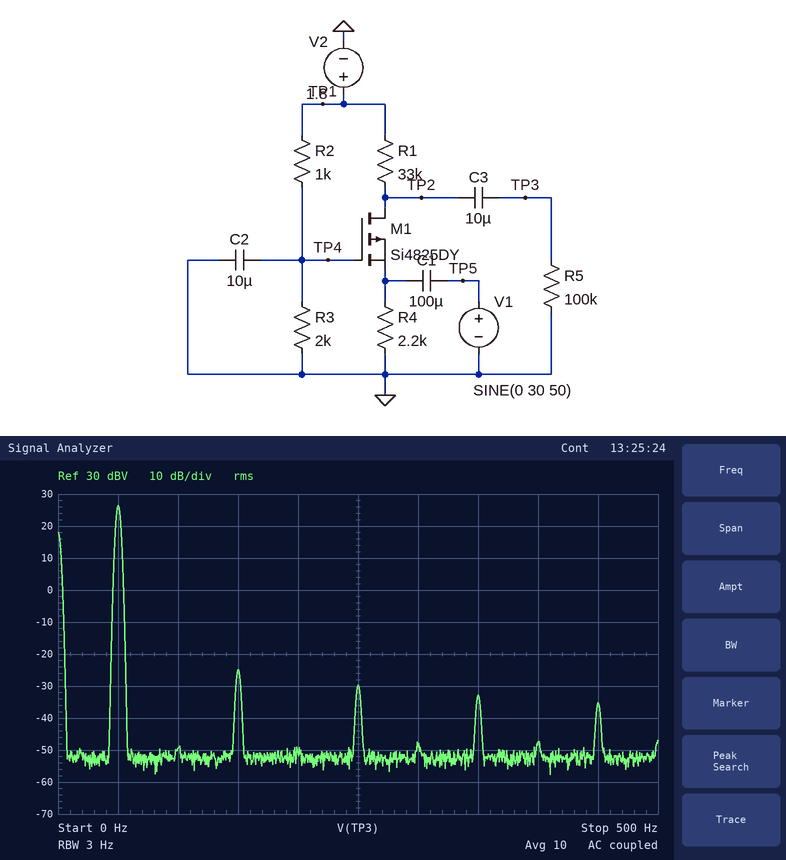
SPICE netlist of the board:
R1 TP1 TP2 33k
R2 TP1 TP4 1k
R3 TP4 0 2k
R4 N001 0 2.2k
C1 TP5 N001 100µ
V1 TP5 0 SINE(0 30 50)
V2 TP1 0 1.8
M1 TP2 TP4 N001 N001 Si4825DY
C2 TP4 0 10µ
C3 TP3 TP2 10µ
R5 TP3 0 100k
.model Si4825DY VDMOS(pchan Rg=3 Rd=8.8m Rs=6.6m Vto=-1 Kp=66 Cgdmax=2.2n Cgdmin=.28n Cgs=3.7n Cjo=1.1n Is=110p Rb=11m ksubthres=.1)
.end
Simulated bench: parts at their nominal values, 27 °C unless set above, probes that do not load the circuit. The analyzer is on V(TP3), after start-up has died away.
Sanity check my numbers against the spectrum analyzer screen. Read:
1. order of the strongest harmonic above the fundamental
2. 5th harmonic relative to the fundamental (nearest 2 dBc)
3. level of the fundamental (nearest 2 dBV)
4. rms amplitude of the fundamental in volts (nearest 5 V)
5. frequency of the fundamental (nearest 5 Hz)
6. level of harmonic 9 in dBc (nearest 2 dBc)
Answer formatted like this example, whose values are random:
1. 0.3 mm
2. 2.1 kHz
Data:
1. 3
2. -56 dBc
3. 26 dBV
4. 20 V
5. 50 Hz
6. -62 dBc
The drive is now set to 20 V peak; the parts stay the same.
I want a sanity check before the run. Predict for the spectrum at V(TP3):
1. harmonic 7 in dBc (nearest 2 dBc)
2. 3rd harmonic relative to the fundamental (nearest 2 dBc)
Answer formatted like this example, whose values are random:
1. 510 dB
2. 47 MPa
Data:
1. -56 dBc
2. -48 dBc
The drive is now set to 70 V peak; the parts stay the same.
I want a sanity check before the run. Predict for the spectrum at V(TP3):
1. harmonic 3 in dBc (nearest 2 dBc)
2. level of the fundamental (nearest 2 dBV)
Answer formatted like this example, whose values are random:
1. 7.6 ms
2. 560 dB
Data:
1. -58 dBc
2. 34 dBV
